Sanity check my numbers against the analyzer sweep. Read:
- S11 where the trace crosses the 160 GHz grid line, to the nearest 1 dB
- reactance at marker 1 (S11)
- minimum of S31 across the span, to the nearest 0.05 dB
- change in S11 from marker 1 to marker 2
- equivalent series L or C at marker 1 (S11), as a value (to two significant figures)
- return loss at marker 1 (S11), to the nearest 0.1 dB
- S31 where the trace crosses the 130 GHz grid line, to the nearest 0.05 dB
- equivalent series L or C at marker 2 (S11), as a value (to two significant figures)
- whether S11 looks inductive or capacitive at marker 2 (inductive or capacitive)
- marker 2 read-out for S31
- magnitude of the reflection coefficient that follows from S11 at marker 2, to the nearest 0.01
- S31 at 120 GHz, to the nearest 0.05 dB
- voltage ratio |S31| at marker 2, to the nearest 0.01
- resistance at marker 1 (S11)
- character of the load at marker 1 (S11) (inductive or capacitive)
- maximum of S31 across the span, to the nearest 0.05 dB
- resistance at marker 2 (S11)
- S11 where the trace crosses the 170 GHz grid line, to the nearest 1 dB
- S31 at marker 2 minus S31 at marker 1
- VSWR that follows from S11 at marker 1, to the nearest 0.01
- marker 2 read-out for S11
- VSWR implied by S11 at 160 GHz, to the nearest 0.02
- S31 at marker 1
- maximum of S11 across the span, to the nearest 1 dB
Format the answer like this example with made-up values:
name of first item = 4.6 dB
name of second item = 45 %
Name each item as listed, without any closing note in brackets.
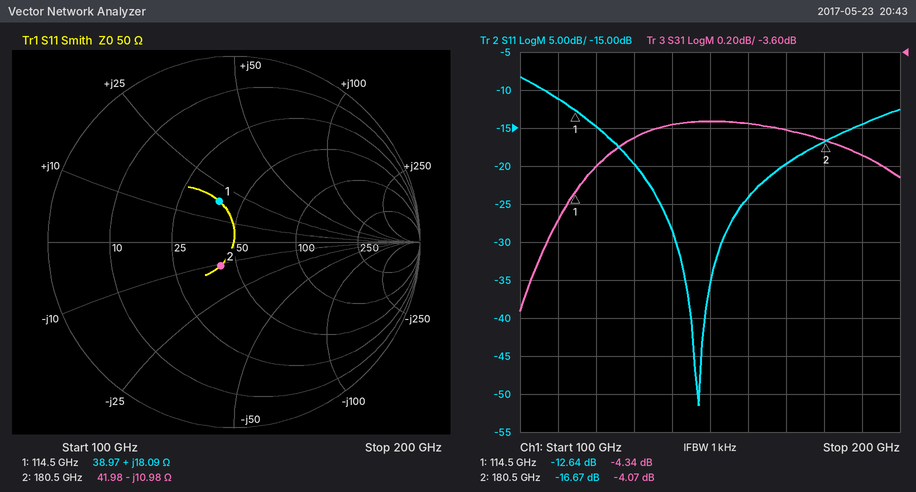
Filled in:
S11 where the trace crosses the 160 GHz grid line, to the nearest 1 dB = -24 dB
reactance at marker 1 = +18.09 Ω
minimum of S31 across the span, to the nearest 0.05 dB = -4.95 dB
change in S11 from marker 1 to marker 2 = -4.03 dB
equivalent series L or C at marker 1 (S11), as a value = 25 pH
return loss at marker 1 (S11), to the nearest 0.1 dB = 12.6 dB
S31 where the trace crosses the 130 GHz grid line, to the nearest 0.05 dB = -4.05 dB
equivalent series L or C at marker 2 (S11), as a value = 80 fF
whether S11 looks inductive or capacitive at marker 2 = capacitive
marker 2 read-out for S31 = -4.07 dB
magnitude of the reflection coefficient that follows from S11 at marker 2, to the nearest 0.01 = 0.15
S31 at 120 GHz, to the nearest 0.05 dB = -4.20 dB
voltage ratio |S31| at marker 2, to the nearest 0.01 = 0.63
resistance at marker 1 = 38.97 Ω
character of the load at marker 1 (S11) = inductive
maximum of S31 across the span, to the nearest 0.05 dB = -3.95 dB
resistance at marker 2 = 41.98 Ω
S11 where the trace crosses the 170 GHz grid line, to the nearest 1 dB = -20 dB
S31 at marker 2 minus S31 at marker 1 = 0.27 dB
VSWR that follows from S11 at marker 1, to the nearest 0.01 = 1.61
marker 2 read-out for S11 = -16.67 dB
VSWR implied by S11 at 160 GHz, to the nearest 0.02 = 1.14
S31 at marker 1 = -4.34 dB
maximum of S11 across the span, to the nearest 1 dB = -8 dB
